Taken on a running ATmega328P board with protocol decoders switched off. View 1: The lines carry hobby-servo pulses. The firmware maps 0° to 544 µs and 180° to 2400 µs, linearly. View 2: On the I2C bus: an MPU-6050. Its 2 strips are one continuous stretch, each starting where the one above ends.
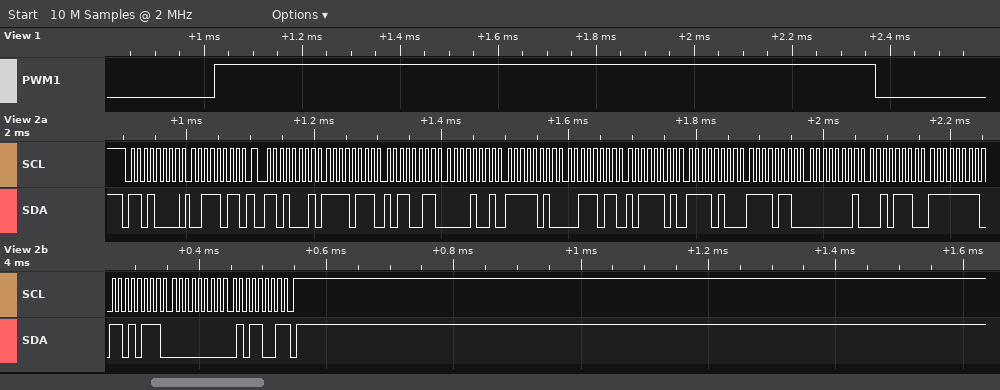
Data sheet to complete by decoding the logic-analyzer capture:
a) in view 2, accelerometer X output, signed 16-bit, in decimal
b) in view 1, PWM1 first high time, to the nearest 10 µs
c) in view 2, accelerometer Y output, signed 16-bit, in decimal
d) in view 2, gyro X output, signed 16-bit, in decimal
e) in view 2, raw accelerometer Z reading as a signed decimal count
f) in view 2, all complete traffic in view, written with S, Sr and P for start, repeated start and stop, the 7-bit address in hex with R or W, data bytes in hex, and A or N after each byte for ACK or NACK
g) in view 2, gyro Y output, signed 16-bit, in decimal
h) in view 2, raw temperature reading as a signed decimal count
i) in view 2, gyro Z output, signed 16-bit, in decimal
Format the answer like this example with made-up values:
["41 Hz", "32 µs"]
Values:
["-2125", "1350 µs", "2554", "302", "15293", "S 68W A 3B A Sr 68R A F7 A B3 A 09 A FA A 3B A BD A F4 A F6 A 01 A 2E A FF A D7 A 00 A 59 N P", "-41", "-2826", "89"]
